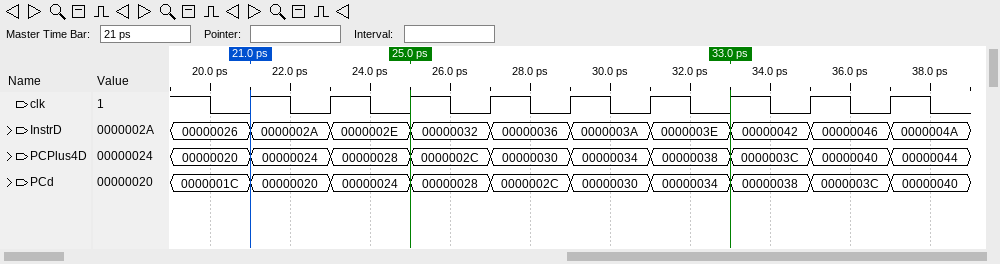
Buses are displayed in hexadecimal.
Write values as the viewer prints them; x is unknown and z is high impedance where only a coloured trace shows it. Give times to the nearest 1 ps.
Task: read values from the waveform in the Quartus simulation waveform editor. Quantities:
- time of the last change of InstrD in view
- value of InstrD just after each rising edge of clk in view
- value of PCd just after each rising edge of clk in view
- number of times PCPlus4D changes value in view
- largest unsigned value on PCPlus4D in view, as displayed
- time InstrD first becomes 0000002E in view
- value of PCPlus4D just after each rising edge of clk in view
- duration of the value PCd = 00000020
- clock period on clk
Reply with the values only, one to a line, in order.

37 ps
0000002A, 0000002E, 00000032, 00000036, 0000003A, 0000003E, 00000042, 00000046, 0000004A
00000020, 00000024, 00000028, 0000002C, 00000030, 00000034, 00000038, 0000003C, 00000040
9
00000044
23 ps
00000024, 00000028, 0000002C, 00000030, 00000034, 00000038, 0000003C, 00000040, 00000044
2 ps
2 ps
